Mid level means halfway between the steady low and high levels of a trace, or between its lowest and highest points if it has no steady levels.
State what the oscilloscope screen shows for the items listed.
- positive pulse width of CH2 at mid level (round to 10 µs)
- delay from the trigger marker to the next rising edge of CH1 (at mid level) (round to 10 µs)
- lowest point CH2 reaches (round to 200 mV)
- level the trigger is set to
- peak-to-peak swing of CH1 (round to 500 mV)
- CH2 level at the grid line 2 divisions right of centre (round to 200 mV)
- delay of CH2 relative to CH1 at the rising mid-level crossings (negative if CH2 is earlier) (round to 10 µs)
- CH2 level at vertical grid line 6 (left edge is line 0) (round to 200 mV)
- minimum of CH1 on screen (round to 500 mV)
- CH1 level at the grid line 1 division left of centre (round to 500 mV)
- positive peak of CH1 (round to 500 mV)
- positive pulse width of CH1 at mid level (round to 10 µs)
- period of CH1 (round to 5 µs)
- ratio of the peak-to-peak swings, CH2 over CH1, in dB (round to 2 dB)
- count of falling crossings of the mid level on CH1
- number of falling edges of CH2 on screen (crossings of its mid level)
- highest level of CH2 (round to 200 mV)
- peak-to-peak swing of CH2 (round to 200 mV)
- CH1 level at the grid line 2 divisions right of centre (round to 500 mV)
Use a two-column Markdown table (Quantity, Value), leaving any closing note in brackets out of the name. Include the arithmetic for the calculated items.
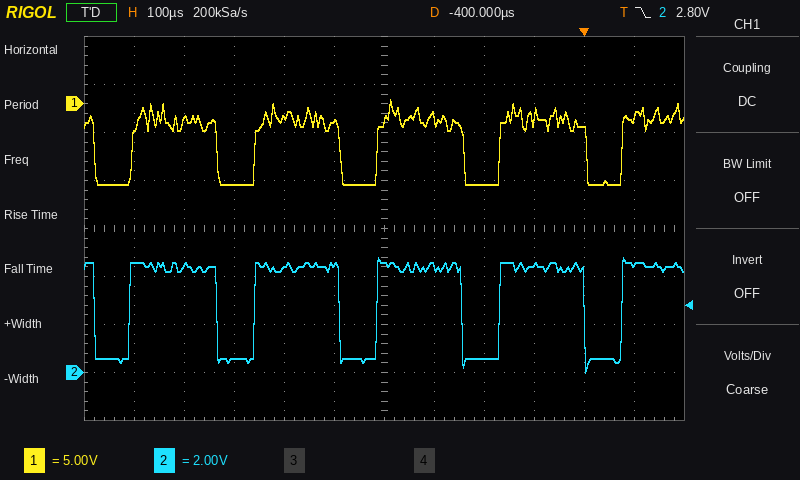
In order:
| Quantity | Value |
|---|---|
| positive pulse width of CH2 at mid level | 170 µs |
| delay from the trigger marker to the next rising edge of CH1 (at mid level) | 80 µs |
| lowest point CH2 reaches | 0.0 V |
| level the trigger is set to | 2.80 V |
| peak-to-peak swing of CH1 | 500 mV − (-8.5 V) = 9.0 V |
| CH2 level at the grid line 2 divisions right of centre | 600 mV |
| delay of CH2 relative to CH1 at the rising mid-level crossings (negative if CH2 is earlier) | 0 µs |
| CH2 level at vertical grid line 6 (left edge is line 0) | 4.6 V |
| minimum of CH1 on screen | -8.5 V |
| CH1 level at the grid line 1 division left of centre | -2.0 V |
| positive peak of CH1 | 500 mV |
| positive pulse width of CH1 at mid level | 170 µs |
| period of CH1 | 245 µs |
| ratio of the peak-to-peak swings, CH2 over CH1, in dB | 20 log10(4.8 V / 9.0 V) ≈ -5.46 dB, so -6 dB to the nearest 2 dB |
| count of falling crossings of the mid level on CH1 | 5 |
| number of falling edges of CH2 on screen | 5 |
| highest level of CH2 | 4.8 V |
| peak-to-peak swing of CH2 | 4.8 V − (0.0 V) = 4.8 V |
| CH1 level at the grid line 2 divisions right of centre | -8.5 V |
